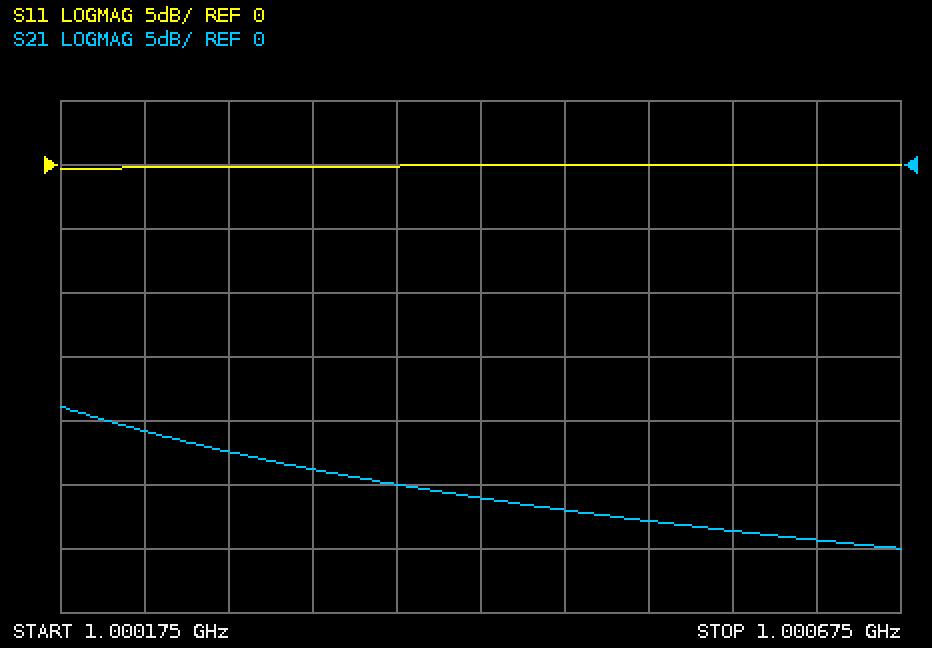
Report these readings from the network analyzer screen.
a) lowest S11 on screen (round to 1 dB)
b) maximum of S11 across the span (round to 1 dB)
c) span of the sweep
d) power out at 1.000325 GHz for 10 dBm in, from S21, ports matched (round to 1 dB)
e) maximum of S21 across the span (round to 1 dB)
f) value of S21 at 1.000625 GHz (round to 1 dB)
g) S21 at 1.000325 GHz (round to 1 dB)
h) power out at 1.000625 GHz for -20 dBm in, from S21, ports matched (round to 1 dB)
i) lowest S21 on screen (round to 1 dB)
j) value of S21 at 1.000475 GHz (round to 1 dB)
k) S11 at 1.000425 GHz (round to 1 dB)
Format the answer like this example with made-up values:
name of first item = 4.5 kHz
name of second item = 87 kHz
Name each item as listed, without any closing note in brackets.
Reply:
lowest S11 on screen = 0 dB
maximum of S11 across the span = 0 dB
span of the sweep = 500 kHz
power out at 1.000325 GHz for 10 dBm in, from S21, ports matched = -14 dBm
maximum of S21 across the span = -19 dB
value of S21 at 1.000625 GHz = -29 dB
S21 at 1.000325 GHz = -24 dB
power out at 1.000625 GHz for -20 dBm in, from S21, ports matched = -49 dBm
lowest S21 on screen = -30 dB
value of S21 at 1.000475 GHz = -27 dB
S11 at 1.000425 GHz = 0 dB
